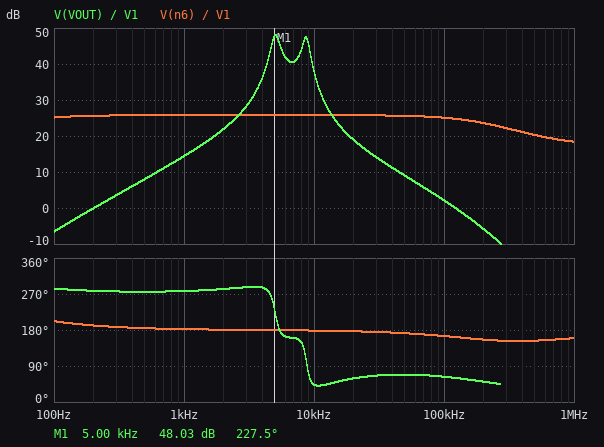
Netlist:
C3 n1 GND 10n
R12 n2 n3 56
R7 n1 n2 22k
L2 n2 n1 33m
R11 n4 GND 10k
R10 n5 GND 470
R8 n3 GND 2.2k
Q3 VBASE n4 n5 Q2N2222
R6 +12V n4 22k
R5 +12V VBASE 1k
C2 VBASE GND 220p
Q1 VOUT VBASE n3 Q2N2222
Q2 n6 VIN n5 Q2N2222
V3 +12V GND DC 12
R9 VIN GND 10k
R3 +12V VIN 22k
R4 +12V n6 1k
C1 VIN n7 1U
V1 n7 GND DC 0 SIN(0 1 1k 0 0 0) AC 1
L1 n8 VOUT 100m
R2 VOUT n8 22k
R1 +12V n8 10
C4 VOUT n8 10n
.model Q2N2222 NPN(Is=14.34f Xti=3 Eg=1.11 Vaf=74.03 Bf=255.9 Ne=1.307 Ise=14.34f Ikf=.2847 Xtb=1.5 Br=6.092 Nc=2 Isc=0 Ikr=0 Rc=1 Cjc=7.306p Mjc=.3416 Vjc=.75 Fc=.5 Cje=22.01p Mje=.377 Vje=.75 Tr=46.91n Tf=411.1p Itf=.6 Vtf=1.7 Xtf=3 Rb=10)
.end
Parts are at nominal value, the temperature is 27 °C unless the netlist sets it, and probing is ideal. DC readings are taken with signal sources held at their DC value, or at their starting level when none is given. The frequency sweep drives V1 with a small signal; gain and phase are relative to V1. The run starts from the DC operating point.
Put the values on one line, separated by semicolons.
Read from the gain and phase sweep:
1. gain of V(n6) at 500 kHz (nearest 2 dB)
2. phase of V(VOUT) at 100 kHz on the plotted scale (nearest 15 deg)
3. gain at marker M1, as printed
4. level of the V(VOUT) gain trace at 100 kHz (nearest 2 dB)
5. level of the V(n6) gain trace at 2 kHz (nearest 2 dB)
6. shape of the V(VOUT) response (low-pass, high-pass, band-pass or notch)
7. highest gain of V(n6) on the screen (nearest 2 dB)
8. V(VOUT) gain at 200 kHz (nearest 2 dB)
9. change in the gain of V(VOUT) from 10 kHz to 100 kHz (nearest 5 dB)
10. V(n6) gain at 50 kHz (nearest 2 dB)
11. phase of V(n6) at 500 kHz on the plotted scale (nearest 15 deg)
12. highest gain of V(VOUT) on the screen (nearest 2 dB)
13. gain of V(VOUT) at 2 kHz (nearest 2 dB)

20 dB; 60 deg; 48.03 dB; 2 dB; 26 dB; band-pass; 26 dB; -6 dB; -35 dB; 26 dB; 150 deg; 48 dB; 22 dB
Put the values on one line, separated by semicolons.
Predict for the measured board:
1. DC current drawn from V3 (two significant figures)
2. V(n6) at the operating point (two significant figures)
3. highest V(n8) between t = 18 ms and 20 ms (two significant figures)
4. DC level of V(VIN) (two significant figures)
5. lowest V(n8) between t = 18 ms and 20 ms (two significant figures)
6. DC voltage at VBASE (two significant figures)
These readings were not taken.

11 mA; 8.9 V; 12 V; 3.6 V; 12 V; 8.9 V
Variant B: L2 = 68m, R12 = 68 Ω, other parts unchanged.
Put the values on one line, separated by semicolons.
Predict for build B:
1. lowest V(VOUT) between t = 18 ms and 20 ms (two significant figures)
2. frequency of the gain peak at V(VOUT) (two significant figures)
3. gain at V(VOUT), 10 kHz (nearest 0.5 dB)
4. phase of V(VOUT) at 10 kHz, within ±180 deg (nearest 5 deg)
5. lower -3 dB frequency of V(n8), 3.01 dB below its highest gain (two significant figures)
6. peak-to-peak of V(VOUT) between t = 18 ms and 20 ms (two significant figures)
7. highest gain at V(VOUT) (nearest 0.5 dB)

3.5 V; 5.2 kHz; 28.0 dB; 60 deg; 5.7 kHz; 19 V; 53.0 dB
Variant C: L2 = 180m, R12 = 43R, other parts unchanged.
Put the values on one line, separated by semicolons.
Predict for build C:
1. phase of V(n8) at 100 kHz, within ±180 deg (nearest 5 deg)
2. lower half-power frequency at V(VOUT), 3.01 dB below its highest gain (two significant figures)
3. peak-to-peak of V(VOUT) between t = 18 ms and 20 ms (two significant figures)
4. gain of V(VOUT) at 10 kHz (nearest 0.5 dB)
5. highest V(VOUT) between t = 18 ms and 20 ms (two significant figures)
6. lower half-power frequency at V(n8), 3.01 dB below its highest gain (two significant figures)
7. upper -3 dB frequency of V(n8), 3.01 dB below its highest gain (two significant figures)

155 deg; 4.5 kHz; 16 V; 26.0 dB; 20 V; 3.4 kHz; 4.2 kHz
